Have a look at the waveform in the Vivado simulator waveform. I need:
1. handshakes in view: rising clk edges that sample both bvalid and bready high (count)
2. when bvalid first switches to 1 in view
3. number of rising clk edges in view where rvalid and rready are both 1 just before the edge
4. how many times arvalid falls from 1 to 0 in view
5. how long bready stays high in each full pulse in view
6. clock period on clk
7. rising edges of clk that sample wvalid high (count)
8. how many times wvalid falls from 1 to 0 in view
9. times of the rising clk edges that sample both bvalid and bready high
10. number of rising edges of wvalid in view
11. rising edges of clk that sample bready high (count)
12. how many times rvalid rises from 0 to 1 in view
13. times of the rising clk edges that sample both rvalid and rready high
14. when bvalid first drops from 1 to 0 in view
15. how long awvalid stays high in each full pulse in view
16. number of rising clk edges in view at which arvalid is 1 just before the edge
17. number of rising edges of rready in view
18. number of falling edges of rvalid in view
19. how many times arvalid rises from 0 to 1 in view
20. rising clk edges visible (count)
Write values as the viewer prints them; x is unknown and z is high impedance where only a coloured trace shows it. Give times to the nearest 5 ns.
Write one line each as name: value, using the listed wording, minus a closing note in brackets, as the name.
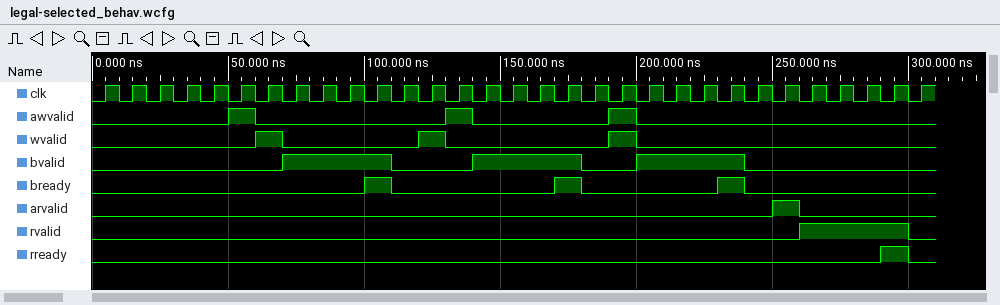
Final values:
handshakes in view: rising clk edges that sample both bvalid and bready high: 3
when bvalid first switches to 1 in view: 70 ns
number of rising clk edges in view where rvalid and rready are both 1 just before the edge: 1
how many times arvalid falls from 1 to 0 in view: 1
how long bready stays high in each full pulse in view: 10 ns, 10 ns, 10 ns
clock period on clk: 10 ns
rising edges of clk that sample wvalid high: 3
how many times wvalid falls from 1 to 0 in view: 3
times of the rising clk edges that sample both bvalid and bready high: 105 ns, 175 ns, 235 ns
number of rising edges of wvalid in view: 3
rising edges of clk that sample bready high: 3
how many times rvalid rises from 0 to 1 in view: 1
times of the rising clk edges that sample both rvalid and rready high: 295 ns
when bvalid first drops from 1 to 0 in view: 110 ns
how long awvalid stays high in each full pulse in view: 10 ns, 10 ns, 10 ns
number of rising clk edges in view at which arvalid is 1 just before the edge: 1
number of rising edges of rready in view: 1
number of falling edges of rvalid in view: 1
how many times arvalid rises from 0 to 1 in view: 1
rising clk edges visible: 31
